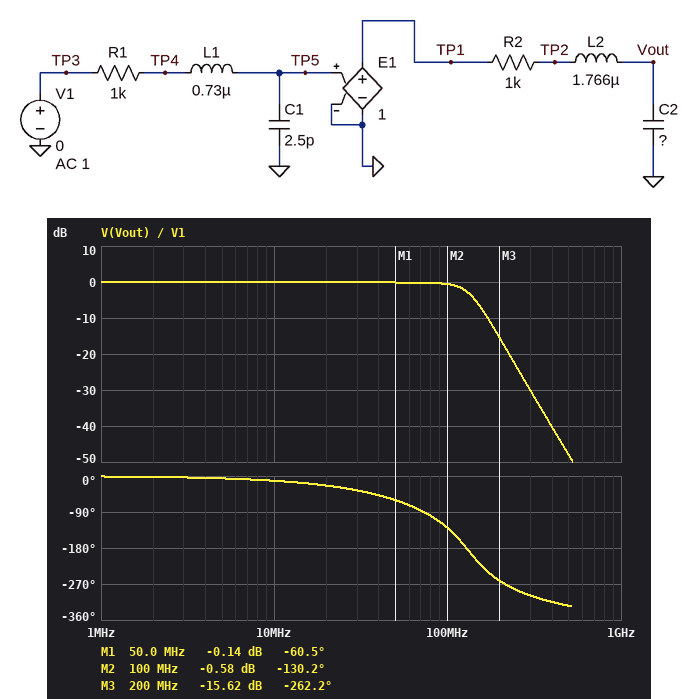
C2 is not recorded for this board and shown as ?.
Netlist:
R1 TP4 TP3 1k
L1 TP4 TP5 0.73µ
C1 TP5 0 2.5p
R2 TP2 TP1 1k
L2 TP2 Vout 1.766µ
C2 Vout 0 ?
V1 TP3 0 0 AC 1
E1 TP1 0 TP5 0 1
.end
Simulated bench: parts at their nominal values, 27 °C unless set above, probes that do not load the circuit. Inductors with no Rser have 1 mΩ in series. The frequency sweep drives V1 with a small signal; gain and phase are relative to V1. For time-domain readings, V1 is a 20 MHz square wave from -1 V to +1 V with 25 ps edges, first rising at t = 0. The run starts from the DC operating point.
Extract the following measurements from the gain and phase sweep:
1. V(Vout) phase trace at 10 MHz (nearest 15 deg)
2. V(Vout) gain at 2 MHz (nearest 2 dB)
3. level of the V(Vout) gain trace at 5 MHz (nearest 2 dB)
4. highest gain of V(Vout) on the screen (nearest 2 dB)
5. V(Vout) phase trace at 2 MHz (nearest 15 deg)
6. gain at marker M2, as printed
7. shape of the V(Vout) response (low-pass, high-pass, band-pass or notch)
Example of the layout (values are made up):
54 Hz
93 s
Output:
-15 deg
0 dB
0 dB
0 dB
0 deg
-0.58 dB
low-pass
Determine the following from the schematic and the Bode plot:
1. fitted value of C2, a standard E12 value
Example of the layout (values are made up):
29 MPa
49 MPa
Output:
820 fF
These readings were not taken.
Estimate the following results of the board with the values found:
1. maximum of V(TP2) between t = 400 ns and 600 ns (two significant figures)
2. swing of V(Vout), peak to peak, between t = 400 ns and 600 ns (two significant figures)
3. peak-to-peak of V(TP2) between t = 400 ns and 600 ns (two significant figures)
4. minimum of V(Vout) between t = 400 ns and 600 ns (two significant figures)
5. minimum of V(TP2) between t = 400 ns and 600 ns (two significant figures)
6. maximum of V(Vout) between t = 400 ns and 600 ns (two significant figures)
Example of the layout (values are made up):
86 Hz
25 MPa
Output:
1.1 V
2.4 V
2.2 V
-1.2 V
-1.1 V
1.2 V
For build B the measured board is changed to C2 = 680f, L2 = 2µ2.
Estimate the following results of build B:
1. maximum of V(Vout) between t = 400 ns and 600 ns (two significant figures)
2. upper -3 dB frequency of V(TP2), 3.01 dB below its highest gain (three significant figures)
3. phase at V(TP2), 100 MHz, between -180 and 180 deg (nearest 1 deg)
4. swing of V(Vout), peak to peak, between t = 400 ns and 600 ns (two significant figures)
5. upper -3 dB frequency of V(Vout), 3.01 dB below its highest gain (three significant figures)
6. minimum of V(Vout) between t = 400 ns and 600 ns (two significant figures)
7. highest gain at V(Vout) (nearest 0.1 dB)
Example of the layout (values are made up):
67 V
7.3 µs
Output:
1.3 V
72.0 MHz
-126 deg
2.6 V
138 MHz
-1.3 V
0.5 dB
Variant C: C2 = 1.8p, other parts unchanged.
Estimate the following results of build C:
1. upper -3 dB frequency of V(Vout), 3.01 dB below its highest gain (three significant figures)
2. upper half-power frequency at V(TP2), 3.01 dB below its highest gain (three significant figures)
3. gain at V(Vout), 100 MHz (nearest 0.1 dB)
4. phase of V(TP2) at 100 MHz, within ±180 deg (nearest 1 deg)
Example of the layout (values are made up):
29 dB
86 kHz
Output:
86.5 MHz
48.0 MHz
-5.3 dB
-3 deg
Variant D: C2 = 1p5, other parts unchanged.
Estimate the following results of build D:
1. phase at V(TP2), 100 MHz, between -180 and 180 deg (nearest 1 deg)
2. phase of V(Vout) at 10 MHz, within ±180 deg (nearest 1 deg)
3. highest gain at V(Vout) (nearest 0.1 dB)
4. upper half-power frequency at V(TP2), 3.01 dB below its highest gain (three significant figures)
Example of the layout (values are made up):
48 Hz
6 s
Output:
7 deg
-14 deg
0.1 dB
53.1 MHz
